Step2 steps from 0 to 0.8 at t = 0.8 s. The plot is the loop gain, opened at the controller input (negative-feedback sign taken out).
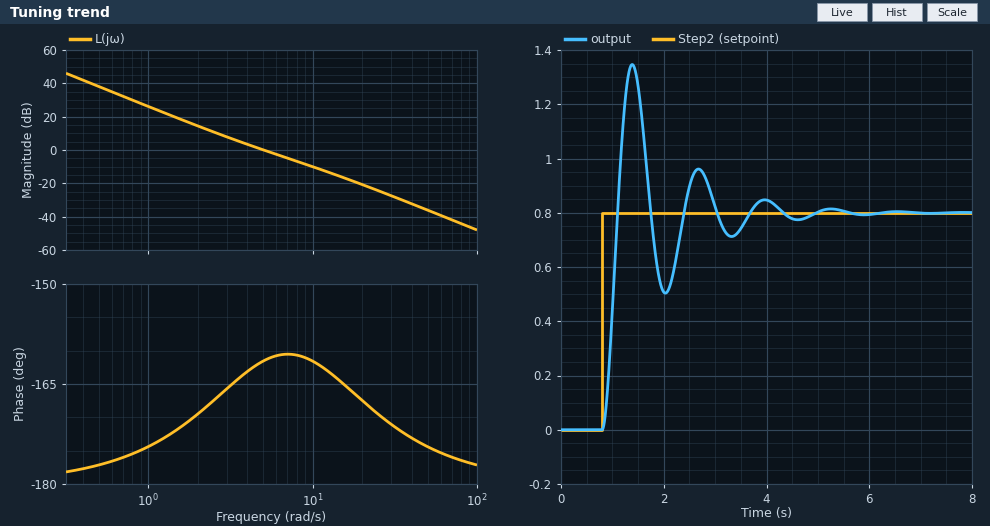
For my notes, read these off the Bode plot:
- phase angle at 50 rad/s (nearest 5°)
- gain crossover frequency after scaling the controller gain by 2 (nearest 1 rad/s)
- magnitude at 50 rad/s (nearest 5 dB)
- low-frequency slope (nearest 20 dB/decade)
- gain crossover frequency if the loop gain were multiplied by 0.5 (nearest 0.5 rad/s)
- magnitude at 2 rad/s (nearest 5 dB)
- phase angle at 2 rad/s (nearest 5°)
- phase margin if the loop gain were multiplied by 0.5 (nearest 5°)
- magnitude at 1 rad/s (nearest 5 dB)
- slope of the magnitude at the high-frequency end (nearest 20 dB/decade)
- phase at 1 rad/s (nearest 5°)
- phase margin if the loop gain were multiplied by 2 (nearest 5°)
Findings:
-175°
8 rad/s
-35 dB
-40 dB/decade
3.5 rad/s
15 dB
-170°
15°
25 dB
-40 dB/decade
-175°
20°
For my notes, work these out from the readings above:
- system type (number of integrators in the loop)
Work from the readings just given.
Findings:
2
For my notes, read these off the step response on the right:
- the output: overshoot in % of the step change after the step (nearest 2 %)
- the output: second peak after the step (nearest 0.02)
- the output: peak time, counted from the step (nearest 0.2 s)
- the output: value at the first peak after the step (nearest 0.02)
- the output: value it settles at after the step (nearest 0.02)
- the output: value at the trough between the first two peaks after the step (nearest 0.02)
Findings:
68 %
0.96
0.6 s
1.34
0.80
0.50
